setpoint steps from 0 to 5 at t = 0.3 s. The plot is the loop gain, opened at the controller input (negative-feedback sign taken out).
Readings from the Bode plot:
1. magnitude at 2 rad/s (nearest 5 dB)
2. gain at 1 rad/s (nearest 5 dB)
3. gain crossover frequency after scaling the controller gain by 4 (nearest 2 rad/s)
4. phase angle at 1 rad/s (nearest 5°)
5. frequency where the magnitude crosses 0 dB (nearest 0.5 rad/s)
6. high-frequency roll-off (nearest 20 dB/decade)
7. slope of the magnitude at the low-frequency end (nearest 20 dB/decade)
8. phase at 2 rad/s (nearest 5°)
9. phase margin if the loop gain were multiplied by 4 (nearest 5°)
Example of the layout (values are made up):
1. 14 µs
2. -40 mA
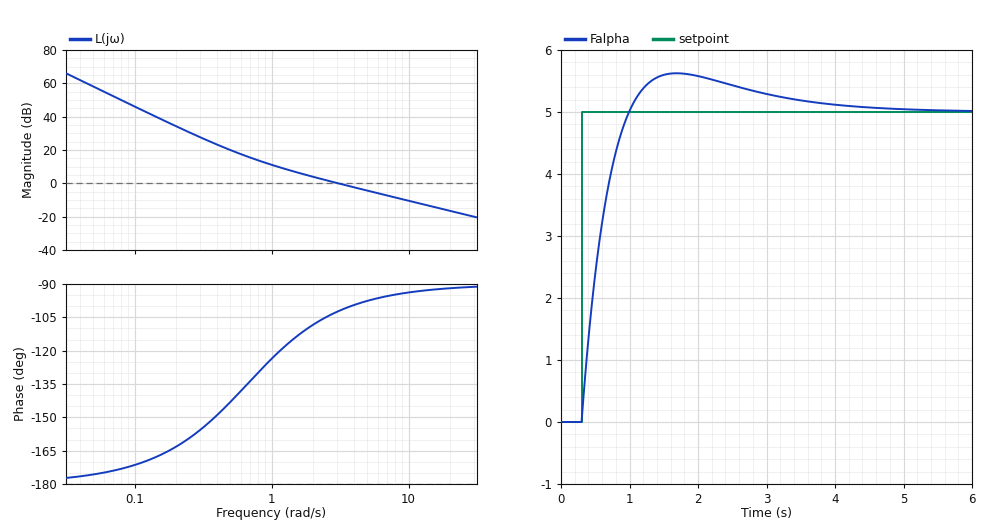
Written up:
1. 5 dB
2. 10 dB
3. 12 rad/s
4. -125°
5. 3.0 rad/s
6. -20 dB/decade
7. -40 dB/decade
8. -110°
9. 85°
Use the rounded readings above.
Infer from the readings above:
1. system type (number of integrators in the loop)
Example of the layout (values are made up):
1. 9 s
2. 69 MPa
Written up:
1. 2
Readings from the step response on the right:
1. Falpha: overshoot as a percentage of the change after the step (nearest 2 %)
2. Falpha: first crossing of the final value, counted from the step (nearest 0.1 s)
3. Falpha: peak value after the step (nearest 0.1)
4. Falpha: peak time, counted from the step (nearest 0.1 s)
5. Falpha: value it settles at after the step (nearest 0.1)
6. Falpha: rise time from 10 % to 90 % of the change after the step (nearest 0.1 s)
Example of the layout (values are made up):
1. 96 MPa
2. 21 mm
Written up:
1. 12 %
2. 0.7 s
3. 5.6
4. 1.4 s
5. 5.0
6. 0.5 s
